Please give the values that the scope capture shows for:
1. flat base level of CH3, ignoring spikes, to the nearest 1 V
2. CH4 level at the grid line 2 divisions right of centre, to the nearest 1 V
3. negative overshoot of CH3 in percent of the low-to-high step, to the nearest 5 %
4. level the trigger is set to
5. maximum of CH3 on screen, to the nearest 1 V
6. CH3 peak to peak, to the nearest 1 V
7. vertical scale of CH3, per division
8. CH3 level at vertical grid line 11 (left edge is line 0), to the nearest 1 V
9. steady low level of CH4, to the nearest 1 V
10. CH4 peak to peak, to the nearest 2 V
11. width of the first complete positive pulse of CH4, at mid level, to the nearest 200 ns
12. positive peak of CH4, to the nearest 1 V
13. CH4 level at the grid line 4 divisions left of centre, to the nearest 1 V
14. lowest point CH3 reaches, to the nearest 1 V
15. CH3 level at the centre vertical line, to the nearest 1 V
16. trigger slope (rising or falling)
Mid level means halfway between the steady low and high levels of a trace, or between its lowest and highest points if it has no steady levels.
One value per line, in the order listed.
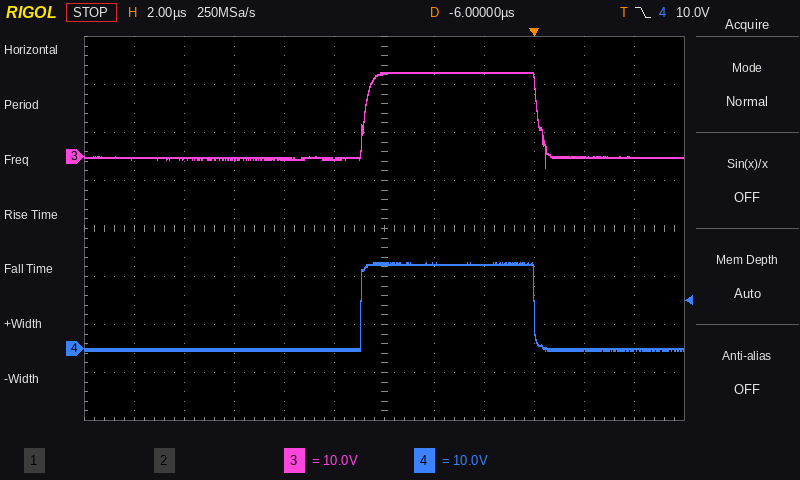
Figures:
0 V
18 V
10 %
10.0 V
18 V
20 V
10 V
0 V
0 V
18 V
7.0 µs
18 V
0 V
-2 V
17 V
falling
